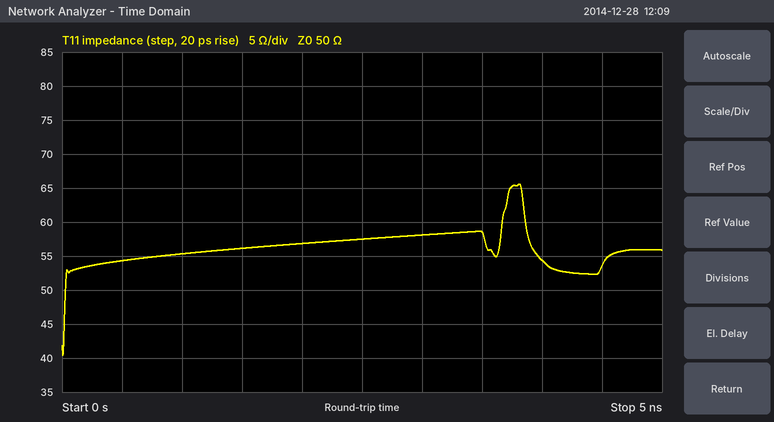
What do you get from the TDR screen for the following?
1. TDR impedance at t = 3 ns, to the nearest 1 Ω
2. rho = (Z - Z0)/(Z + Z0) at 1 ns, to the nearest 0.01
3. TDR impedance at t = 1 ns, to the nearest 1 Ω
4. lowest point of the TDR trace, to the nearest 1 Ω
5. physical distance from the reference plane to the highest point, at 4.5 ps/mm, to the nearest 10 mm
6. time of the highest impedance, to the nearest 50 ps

58 Ω
+0.05
55 Ω
40 Ω
420 mm
3.80 ns
